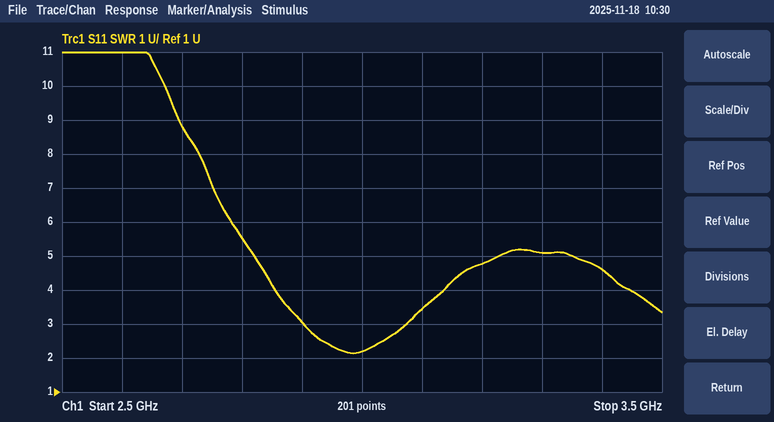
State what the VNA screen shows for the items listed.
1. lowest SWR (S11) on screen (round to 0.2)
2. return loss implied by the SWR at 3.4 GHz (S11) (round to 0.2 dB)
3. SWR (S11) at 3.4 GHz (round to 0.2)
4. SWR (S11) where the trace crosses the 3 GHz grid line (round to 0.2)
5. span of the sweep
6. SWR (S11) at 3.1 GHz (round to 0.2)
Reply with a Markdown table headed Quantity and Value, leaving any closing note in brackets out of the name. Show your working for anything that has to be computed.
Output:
| Quantity | Value |
|---|---|
| lowest SWR (S11) on screen | 2.2 |
| return loss implied by the SWR at 3.4 GHz (S11) | −20 log10((4.6 − 1)/(4.6 + 1)) ≈ 3.8 dB |
| SWR (S11) at 3.4 GHz | 4.6 |
| SWR (S11) where the trace crosses the 3 GHz grid line | 2.2 |
| span of the sweep | 1 GHz |
| SWR (S11) at 3.1 GHz | 3.4 |
